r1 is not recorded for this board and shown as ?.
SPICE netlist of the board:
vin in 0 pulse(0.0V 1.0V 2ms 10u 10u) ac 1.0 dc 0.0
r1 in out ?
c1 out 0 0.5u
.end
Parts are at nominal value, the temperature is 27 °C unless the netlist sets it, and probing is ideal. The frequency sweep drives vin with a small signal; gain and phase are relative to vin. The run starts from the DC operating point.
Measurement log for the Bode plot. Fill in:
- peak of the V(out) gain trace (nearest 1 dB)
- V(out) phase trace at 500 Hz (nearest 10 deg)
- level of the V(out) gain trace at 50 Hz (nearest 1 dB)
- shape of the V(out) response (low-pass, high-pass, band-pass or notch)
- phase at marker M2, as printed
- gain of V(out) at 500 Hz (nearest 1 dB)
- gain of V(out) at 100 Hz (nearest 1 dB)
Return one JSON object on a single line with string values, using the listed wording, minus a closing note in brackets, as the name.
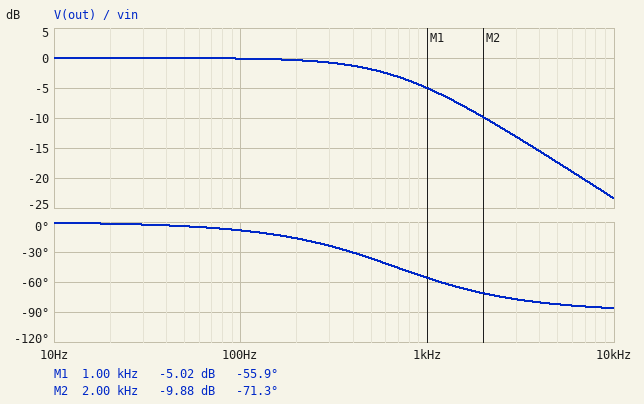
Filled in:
{"peak of the V(out) gain trace": "0 dB", "V(out) phase trace at 500 Hz": "-40 deg", "level of the V(out) gain trace at 50 Hz": "0 dB", "shape of the V(out) response": "low-pass", "phase at marker M2, as printed": "-71.3 deg", "gain of V(out) at 500 Hz": "-2 dB", "gain of V(out) at 100 Hz": "0 dB"}
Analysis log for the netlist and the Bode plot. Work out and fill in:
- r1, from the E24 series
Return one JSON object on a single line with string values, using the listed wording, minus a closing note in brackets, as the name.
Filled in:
{"r1, from the E24 series": "470 Ω"}
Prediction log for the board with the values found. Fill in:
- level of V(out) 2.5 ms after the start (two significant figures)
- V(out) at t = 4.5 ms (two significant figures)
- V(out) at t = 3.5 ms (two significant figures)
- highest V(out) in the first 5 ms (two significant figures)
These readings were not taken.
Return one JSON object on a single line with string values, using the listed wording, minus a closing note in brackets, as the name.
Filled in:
{"level of V(out) 2.5 ms after the start": "880 mV", "V(out) at t = 4.5 ms": "1.0 V", "V(out) at t = 3.5 ms": "1.0 V", "highest V(out) in the first 5 ms": "1.0 V"}
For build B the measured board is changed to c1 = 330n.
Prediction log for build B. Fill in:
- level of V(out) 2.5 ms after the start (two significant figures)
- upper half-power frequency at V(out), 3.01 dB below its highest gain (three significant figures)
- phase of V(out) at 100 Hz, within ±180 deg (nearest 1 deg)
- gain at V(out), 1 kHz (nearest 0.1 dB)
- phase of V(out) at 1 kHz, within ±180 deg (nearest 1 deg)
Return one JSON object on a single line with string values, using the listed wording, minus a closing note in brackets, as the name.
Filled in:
{"level of V(out) 2.5 ms after the start": "960 mV", "upper half-power frequency at V(out), 3.01 dB below its highest gain": "1.03 kHz", "phase of V(out) at 100 Hz, within ±180 deg": "-6 deg", "gain at V(out), 1 kHz": "-2.9 dB", "phase of V(out) at 1 kHz, within ±180 deg": "-44 deg"}
